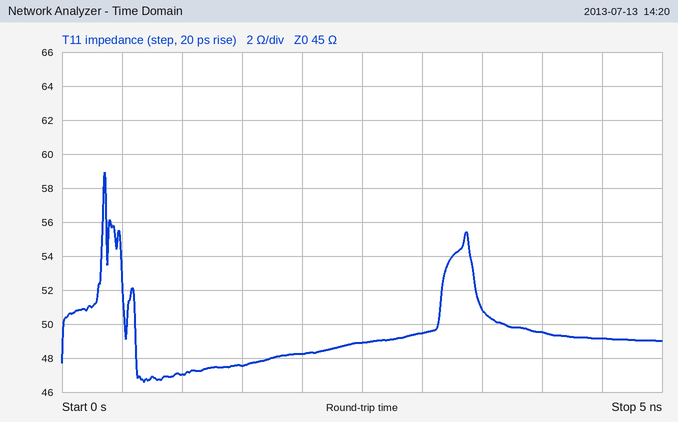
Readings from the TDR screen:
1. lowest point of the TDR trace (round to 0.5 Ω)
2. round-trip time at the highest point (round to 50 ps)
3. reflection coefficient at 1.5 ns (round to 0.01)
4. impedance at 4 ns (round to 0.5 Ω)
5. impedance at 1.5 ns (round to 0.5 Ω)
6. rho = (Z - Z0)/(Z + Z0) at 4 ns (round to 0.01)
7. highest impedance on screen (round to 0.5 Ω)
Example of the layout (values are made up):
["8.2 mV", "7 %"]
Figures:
["46.5 Ω", "350 ps", "+0.03", "49.5 Ω", "47.5 Ω", "+0.05", "59.0 Ω"]
